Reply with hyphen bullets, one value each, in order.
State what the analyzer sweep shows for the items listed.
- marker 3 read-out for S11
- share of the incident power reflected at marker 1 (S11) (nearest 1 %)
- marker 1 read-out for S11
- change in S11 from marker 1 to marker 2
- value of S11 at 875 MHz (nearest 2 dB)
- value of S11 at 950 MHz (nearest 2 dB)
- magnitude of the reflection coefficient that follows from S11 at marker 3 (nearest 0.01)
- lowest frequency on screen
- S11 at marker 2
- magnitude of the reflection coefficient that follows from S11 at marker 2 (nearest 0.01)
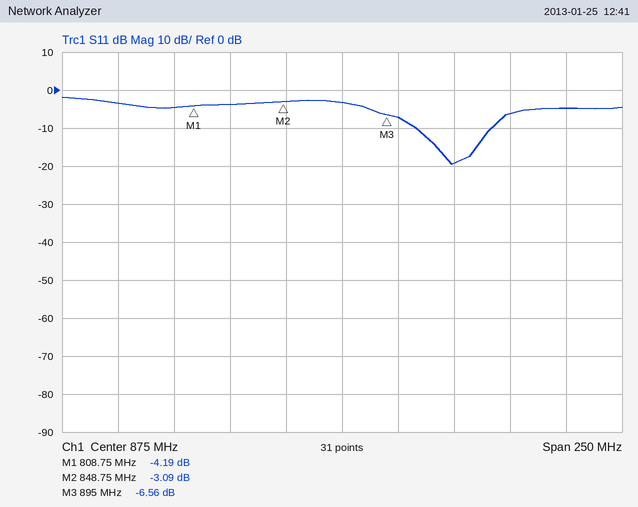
- -6.56 dB
- 38 %
- -4.19 dB
- 1.10 dB
- -4 dB
- -6 dB
- 0.47
- 750 MHz
- -3.09 dB
- 0.70
